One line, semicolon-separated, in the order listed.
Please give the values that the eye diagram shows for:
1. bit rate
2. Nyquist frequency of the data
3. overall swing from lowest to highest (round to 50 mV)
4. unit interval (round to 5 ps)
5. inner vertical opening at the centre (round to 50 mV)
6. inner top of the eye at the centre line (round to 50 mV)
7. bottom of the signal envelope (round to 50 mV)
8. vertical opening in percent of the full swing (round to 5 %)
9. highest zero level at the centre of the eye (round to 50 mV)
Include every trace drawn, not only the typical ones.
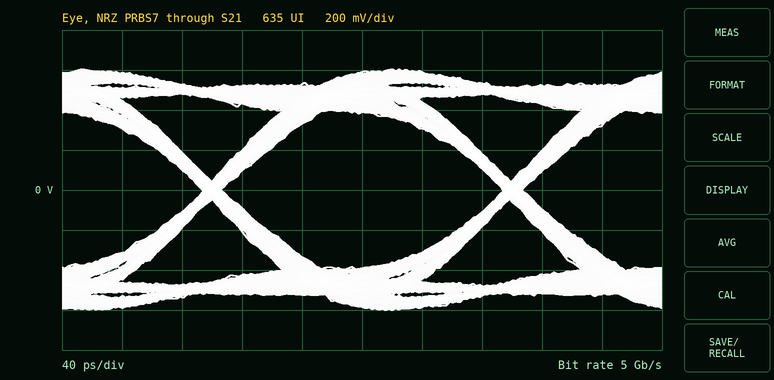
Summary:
5 Gb/s; 2.5 GHz; 1.20 V; 200 ps; 800 mV; 400 mV; -600 mV; 65 %; -400 mV
